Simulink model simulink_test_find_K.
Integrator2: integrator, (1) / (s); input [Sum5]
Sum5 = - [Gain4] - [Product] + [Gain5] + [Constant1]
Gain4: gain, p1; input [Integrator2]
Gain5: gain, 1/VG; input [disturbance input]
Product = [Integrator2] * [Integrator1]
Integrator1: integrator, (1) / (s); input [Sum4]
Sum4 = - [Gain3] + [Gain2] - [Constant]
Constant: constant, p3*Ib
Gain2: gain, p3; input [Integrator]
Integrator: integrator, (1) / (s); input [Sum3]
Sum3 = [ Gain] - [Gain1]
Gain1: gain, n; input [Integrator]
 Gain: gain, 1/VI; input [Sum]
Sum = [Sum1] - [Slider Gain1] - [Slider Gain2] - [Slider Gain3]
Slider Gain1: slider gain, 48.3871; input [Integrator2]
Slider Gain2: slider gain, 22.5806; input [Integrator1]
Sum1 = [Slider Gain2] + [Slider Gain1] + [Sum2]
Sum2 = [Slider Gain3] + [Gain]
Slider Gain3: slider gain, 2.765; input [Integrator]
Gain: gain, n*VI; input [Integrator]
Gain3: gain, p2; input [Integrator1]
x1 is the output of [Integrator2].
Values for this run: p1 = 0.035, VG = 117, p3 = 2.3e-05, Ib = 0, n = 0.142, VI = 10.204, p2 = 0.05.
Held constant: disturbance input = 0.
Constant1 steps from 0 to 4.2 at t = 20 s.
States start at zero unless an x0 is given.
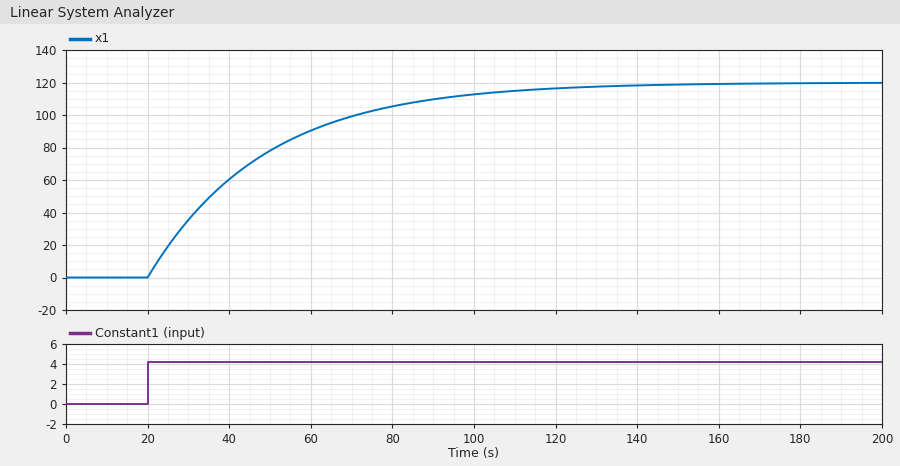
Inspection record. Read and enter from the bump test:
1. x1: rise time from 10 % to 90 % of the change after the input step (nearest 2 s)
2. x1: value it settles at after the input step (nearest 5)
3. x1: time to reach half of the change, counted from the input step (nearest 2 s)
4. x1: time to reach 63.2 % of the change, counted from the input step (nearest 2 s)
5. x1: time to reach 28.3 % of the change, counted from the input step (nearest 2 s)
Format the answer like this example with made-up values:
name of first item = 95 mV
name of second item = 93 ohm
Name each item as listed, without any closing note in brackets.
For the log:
x1: rise time from 10 % to 90 % of the change after the input step = 62 s
x1: value it settles at after the input step = 120
x1: time to reach half of the change, counted from the input step = 20 s
x1: time to reach 63.2 % of the change, counted from the input step = 28 s
x1: time to reach 28.3 % of the change, counted from the input step = 10 s
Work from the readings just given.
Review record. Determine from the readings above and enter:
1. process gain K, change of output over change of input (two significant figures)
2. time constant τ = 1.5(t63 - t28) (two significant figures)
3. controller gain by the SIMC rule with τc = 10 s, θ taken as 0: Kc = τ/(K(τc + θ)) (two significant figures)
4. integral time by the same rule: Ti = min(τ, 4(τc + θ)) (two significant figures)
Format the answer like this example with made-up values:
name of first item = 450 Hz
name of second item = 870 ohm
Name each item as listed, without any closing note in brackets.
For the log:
process gain K, change of output over change of input = 29
time constant τ = 1.5(t63 - t28) = 27 s
controller gain by the SIMC rule with τc = 10 s, θ taken as 0: Kc = τ/(K(τc + θ)) = 0.093
integral time by the same rule: Ti = min(τ, 4(τc + θ)) = 27 s
